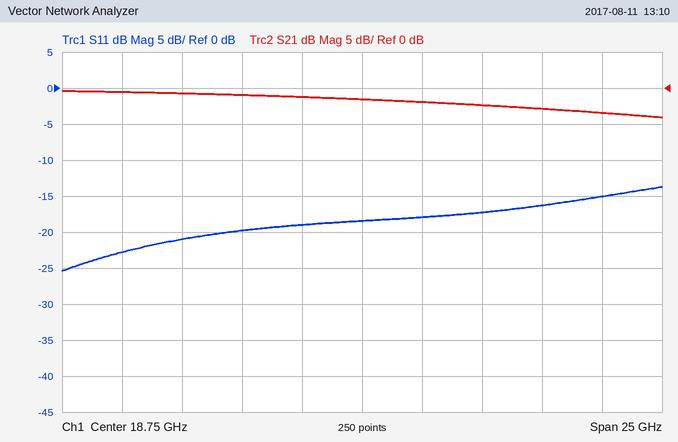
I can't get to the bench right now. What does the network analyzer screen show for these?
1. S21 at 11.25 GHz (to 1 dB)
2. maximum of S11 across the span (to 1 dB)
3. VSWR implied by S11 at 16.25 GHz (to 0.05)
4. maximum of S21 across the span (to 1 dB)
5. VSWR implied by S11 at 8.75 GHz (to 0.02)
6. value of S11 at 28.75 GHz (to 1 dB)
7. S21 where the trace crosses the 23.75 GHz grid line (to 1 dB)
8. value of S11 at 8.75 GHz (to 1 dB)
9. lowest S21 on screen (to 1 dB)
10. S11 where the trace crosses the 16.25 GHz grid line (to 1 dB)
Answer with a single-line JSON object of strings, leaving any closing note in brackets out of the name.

{"S21 at 11.25 GHz": "-1 dB", "maximum of S11 across the span": "-14 dB", "VSWR implied by S11 at 16.25 GHz": "1.25", "maximum of S21 across the span": "0 dB", "VSWR implied by S11 at 8.75 GHz": "1.16", "value of S11 at 28.75 GHz": "-15 dB", "S21 where the trace crosses the 23.75 GHz grid line": "-2 dB", "value of S11 at 8.75 GHz": "-23 dB", "lowest S21 on screen": "-4 dB", "S11 where the trace crosses the 16.25 GHz grid line": "-19 dB"}
